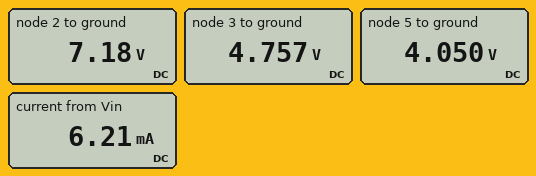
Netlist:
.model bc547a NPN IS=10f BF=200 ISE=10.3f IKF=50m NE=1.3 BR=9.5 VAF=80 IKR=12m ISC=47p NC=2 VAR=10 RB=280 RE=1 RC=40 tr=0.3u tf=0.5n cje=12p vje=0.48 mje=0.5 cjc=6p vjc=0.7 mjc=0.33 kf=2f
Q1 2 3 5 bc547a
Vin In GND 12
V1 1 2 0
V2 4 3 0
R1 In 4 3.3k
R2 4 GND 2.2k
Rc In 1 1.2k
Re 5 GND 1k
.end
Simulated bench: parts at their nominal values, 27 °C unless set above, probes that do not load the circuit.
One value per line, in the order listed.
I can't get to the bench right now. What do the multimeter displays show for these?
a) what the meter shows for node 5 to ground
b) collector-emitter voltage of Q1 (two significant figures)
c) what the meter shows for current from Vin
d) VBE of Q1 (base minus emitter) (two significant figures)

4.050 V
3.1 V
6.21 mA
710 mV
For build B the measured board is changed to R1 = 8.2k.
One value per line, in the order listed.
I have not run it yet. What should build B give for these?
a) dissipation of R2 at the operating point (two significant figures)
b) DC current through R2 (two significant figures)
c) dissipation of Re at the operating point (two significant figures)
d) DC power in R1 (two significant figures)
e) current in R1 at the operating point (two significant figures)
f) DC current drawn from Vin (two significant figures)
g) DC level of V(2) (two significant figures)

2.9 mW
1.1 mA
3.4 mW
11 mW
1.2 mA
3.0 mA
9.8 V
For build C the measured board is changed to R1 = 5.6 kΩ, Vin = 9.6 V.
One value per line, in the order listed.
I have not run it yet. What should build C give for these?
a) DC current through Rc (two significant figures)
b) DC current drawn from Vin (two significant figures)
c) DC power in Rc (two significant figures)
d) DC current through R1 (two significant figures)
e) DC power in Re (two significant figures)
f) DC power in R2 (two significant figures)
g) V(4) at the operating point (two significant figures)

2.0 mA
3.2 mA
4.7 mW
1.2 mA
4.0 mW
3.3 mW
2.7 V
